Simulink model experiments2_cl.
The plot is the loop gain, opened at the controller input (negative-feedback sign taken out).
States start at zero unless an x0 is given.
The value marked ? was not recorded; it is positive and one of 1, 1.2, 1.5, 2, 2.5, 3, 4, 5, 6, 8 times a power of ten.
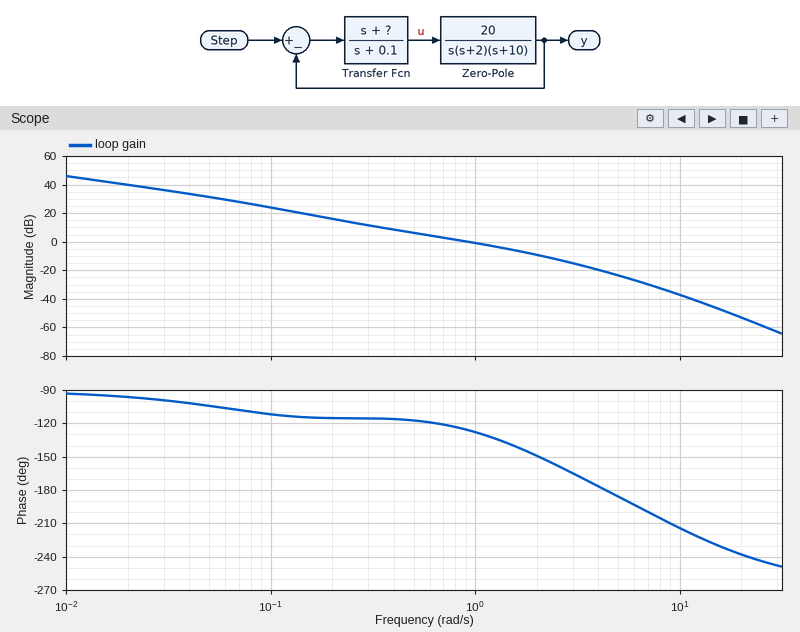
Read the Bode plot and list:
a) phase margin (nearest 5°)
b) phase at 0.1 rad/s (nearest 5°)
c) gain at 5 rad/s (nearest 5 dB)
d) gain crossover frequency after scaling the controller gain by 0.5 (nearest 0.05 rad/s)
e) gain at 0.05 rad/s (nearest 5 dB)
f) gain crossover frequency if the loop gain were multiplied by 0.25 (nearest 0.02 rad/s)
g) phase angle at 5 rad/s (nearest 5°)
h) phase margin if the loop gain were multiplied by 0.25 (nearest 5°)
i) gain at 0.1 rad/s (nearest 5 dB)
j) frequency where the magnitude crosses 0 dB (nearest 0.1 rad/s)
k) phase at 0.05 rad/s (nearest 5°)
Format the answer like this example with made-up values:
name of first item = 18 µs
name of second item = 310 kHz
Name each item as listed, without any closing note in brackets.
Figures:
phase margin = 55°
phase at 0.1 rad/s = -110°
gain at 5 rad/s = -25 dB
gain crossover frequency after scaling the controller gain by 0.5 = 0.50 rad/s
gain at 0.05 rad/s = 30 dB
gain crossover frequency if the loop gain were multiplied by 0.25 = 0.28 rad/s
phase angle at 5 rad/s = -185°
phase margin if the loop gain were multiplied by 0.25 = 65°
gain at 0.1 rad/s = 25 dB
frequency where the magnitude crosses 0 dB = 0.9 rad/s
phase at 0.05 rad/s = -105°
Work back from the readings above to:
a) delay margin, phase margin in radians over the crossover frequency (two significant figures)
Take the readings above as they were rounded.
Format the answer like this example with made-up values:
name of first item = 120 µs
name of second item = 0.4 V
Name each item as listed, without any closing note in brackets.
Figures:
delay margin, phase margin in radians over the crossover frequency = 1.1 s
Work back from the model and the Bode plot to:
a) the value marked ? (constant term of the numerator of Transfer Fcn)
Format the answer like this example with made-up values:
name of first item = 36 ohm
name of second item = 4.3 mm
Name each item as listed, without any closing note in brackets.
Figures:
the value marked ? = 0.2
